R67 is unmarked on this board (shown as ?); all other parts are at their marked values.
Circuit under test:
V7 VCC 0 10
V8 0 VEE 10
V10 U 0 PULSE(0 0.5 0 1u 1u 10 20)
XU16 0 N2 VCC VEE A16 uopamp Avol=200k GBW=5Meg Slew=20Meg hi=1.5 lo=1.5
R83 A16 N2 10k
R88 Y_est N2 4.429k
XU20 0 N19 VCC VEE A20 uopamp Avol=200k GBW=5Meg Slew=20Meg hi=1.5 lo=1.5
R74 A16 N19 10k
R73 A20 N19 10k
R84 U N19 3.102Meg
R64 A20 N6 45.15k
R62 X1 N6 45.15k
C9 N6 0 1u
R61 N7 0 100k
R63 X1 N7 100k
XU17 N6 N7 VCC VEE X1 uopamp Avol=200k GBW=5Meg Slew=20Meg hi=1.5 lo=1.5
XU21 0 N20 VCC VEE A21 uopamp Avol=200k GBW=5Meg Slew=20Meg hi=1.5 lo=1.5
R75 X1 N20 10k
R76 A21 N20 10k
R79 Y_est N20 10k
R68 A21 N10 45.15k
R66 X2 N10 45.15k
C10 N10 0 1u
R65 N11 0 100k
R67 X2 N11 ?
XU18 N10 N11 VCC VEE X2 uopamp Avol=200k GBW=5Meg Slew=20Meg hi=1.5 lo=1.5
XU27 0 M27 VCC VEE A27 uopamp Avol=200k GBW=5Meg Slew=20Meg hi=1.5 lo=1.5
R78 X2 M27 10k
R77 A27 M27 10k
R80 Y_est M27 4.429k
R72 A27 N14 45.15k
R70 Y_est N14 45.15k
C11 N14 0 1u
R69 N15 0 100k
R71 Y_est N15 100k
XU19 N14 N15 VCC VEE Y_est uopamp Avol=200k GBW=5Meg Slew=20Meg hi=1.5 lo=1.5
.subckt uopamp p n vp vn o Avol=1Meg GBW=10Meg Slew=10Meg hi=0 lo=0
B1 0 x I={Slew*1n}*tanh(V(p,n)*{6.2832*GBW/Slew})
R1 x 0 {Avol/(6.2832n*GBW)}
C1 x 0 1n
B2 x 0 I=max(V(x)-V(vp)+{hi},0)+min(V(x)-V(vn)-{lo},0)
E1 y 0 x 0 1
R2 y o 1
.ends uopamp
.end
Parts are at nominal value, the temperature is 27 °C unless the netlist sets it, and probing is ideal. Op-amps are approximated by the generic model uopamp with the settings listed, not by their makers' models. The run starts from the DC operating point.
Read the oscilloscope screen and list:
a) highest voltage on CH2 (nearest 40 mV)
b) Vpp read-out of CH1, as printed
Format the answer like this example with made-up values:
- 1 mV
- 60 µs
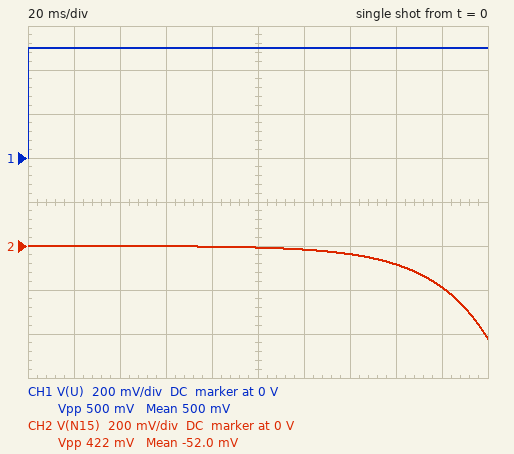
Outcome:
- 0 V
- 500 mV
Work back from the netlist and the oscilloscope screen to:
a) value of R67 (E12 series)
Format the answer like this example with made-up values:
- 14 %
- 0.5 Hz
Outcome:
- 82 kΩ
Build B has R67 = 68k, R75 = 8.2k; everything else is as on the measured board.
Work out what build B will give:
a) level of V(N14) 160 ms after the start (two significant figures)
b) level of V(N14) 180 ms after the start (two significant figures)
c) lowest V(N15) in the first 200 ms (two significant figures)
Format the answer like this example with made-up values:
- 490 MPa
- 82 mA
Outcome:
- -89 mV
- -200 mV
- -450 mV
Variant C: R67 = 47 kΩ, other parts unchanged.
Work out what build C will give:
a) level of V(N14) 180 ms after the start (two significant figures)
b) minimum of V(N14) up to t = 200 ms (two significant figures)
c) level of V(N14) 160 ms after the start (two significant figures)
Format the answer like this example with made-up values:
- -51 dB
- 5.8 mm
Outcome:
- -54 mV
- -100 mV
- -28 mV
